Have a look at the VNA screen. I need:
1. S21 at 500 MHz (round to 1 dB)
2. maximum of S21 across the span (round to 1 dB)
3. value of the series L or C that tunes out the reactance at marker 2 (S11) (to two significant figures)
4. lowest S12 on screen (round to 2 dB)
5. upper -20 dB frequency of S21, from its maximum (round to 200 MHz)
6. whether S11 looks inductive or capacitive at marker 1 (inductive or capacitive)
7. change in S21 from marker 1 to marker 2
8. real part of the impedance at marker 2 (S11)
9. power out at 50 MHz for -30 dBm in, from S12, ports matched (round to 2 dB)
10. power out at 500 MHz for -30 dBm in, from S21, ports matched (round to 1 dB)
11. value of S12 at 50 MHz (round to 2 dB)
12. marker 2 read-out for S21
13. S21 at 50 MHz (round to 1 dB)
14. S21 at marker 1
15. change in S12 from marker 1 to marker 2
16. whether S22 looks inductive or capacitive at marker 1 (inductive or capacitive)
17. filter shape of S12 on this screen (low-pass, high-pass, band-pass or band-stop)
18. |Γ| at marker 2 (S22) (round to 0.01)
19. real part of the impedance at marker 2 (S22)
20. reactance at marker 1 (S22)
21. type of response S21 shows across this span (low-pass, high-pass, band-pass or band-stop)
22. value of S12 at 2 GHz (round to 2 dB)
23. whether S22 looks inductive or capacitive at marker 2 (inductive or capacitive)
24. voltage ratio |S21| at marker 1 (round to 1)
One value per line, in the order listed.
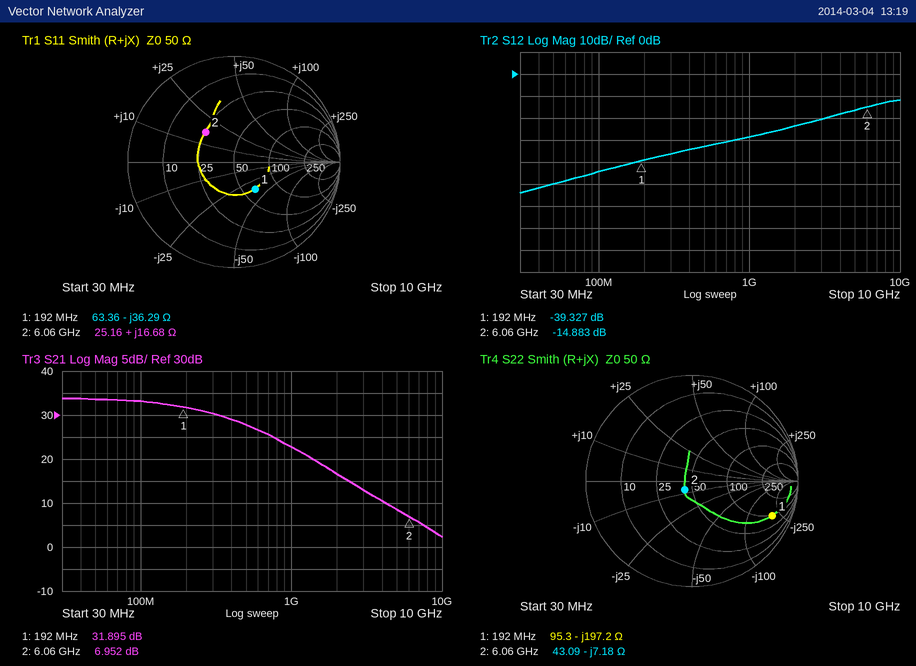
28 dB
34 dB
1.6 pF
-54 dB
2.8 GHz
capacitive
-24.943 dB
25.16 Ω
-80 dBm
-2 dBm
-50 dB
6.952 dB
34 dB
31.895 dB
24.444 dB
capacitive
high-pass
0.11
43.09 Ω
-197.2 Ω
low-pass
-24 dB
capacitive
39
